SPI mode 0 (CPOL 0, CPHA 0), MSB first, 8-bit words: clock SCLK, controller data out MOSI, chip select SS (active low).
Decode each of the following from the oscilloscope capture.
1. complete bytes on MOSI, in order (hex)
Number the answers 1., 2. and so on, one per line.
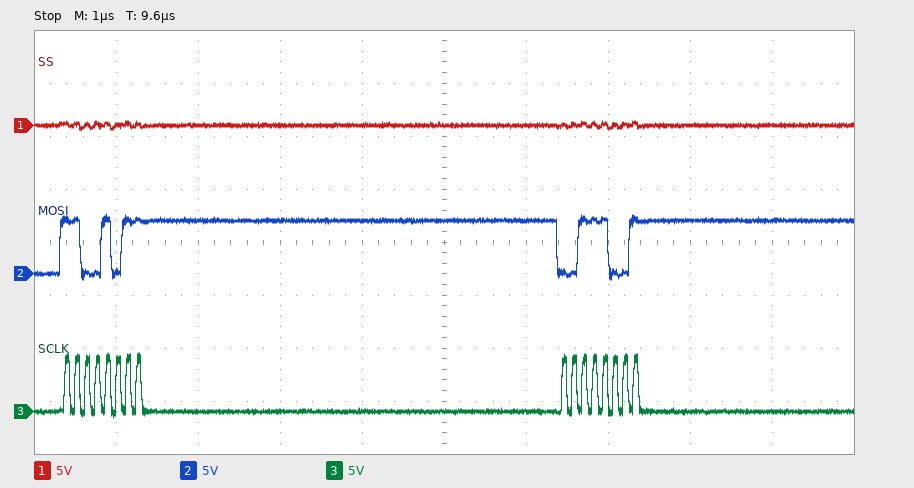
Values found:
1. 0xCB 0x39
